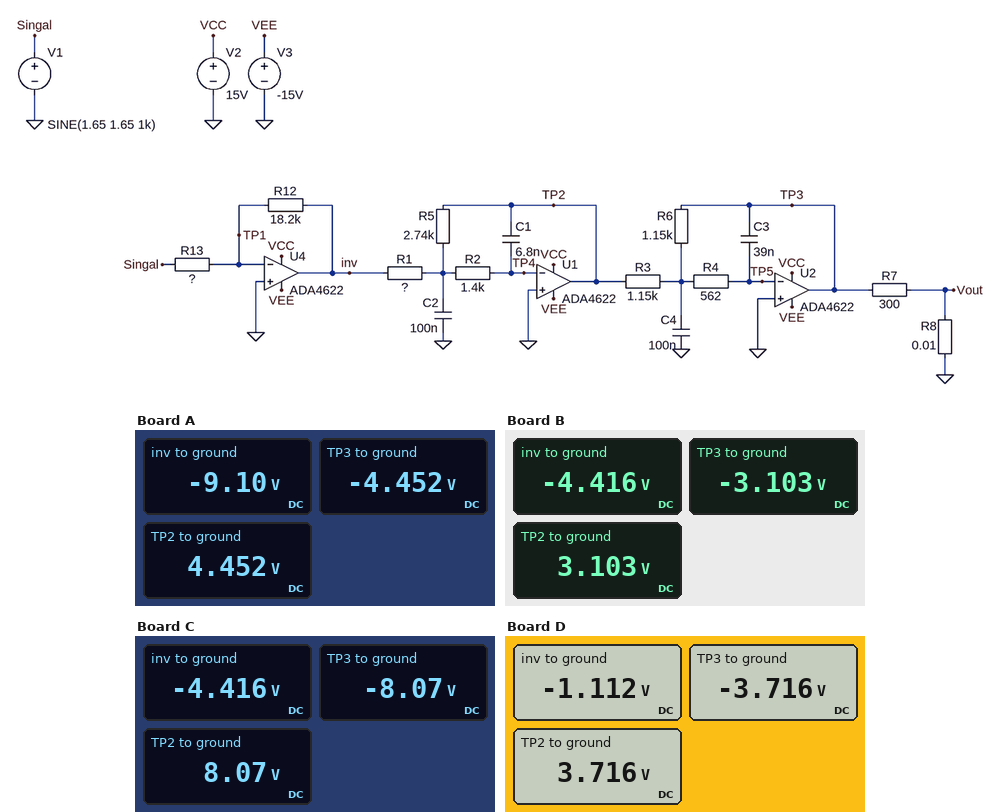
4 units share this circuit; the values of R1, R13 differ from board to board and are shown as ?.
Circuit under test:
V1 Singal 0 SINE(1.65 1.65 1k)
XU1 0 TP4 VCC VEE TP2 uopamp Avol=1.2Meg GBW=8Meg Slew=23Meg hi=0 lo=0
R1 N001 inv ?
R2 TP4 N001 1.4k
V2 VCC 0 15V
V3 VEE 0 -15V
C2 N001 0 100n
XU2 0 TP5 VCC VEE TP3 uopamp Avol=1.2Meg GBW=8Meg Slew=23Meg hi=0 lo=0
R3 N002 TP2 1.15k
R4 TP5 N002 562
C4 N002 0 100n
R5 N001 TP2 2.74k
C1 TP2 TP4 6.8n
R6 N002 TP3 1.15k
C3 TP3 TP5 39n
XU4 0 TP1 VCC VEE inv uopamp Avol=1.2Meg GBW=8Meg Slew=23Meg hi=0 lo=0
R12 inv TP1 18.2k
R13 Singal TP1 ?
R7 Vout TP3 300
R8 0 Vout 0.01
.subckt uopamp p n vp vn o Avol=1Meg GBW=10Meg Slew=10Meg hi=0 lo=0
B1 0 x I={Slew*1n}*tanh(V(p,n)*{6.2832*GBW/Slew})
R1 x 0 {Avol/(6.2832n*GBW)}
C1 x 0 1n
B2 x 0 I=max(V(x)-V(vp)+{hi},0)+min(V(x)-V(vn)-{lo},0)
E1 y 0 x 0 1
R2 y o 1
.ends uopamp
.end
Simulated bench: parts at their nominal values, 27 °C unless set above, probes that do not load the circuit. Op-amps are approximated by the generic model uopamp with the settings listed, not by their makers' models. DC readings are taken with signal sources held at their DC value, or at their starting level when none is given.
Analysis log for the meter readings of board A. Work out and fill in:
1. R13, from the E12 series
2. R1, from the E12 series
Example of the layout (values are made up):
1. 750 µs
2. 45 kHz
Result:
1. 3.3 kΩ
2. 5.6 kΩ
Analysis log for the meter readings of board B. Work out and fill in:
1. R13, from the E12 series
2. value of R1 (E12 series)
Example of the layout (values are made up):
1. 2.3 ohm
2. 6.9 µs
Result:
1. 6.8 kΩ
2. 3.9 kΩ
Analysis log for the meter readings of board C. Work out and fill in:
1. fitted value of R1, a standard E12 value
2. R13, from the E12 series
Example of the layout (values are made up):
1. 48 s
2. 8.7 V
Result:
1. 1.5 kΩ
2. 6.8 kΩ
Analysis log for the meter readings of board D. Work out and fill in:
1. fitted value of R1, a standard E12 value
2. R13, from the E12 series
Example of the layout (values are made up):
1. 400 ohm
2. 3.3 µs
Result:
1. 820 Ω
2. 27 kΩ
